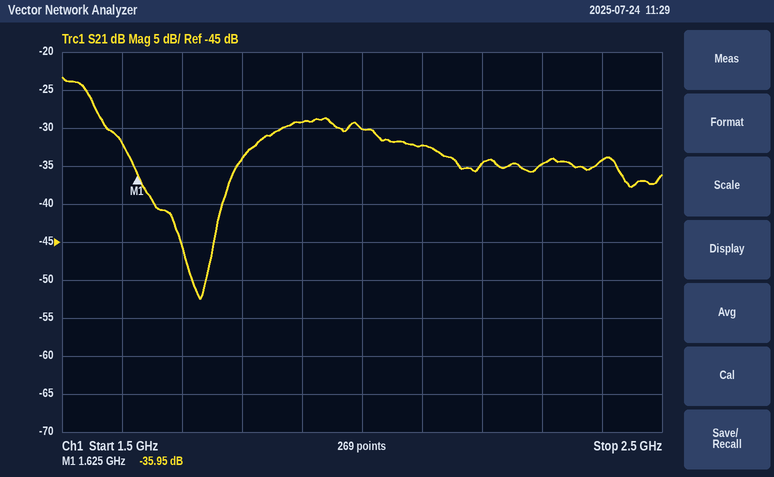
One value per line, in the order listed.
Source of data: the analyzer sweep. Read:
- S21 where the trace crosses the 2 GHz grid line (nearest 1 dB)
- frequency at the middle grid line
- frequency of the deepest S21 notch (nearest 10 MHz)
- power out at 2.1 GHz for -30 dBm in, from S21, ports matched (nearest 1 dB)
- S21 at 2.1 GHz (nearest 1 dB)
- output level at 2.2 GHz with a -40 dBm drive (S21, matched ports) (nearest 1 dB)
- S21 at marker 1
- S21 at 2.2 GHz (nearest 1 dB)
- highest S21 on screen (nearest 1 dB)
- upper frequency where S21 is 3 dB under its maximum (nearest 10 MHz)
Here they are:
-30 dB
2 GHz
1.73 GHz
-62 dBm
-32 dB
-75 dBm
-35.95 dB
-35 dB
-23 dB
1.55 GHz
